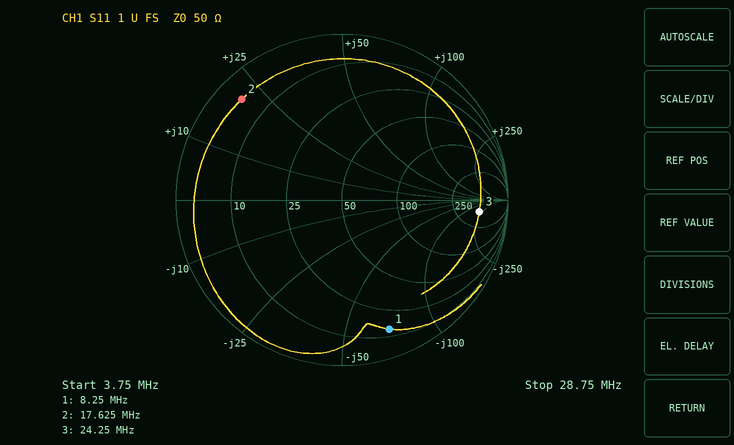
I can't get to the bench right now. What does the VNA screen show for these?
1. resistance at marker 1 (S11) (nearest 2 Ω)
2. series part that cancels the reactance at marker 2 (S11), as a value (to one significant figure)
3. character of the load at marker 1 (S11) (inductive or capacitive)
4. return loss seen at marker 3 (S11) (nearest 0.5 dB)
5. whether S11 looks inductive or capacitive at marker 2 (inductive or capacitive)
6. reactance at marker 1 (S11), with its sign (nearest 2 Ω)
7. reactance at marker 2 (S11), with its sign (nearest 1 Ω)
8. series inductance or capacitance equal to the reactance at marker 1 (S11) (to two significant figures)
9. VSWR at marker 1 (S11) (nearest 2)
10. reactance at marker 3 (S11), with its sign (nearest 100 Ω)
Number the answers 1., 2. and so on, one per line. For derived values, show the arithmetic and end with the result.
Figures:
1. 14 Ω
2. C = 1/(2π × 17.625 MHz × 21 Ω) ≈ 430 pF, so 400 pF to one significant figure
3. capacitive
4. 1.5 dB
5. inductive
6. -70 Ω
7. +21 Ω
8. C = 1/(2π × 8.25 MHz × 70 Ω) ≈ 276 pF, so 280 pF to two significant figures
9. 10
10. -200 Ω
